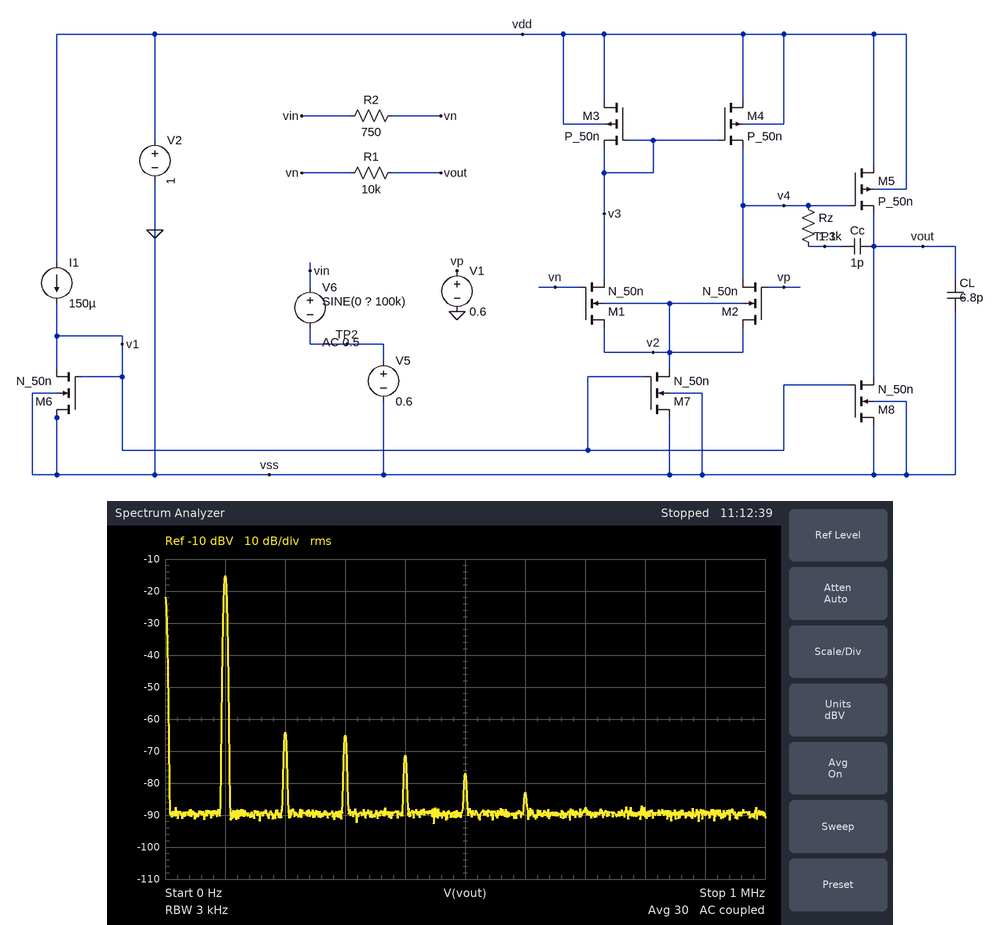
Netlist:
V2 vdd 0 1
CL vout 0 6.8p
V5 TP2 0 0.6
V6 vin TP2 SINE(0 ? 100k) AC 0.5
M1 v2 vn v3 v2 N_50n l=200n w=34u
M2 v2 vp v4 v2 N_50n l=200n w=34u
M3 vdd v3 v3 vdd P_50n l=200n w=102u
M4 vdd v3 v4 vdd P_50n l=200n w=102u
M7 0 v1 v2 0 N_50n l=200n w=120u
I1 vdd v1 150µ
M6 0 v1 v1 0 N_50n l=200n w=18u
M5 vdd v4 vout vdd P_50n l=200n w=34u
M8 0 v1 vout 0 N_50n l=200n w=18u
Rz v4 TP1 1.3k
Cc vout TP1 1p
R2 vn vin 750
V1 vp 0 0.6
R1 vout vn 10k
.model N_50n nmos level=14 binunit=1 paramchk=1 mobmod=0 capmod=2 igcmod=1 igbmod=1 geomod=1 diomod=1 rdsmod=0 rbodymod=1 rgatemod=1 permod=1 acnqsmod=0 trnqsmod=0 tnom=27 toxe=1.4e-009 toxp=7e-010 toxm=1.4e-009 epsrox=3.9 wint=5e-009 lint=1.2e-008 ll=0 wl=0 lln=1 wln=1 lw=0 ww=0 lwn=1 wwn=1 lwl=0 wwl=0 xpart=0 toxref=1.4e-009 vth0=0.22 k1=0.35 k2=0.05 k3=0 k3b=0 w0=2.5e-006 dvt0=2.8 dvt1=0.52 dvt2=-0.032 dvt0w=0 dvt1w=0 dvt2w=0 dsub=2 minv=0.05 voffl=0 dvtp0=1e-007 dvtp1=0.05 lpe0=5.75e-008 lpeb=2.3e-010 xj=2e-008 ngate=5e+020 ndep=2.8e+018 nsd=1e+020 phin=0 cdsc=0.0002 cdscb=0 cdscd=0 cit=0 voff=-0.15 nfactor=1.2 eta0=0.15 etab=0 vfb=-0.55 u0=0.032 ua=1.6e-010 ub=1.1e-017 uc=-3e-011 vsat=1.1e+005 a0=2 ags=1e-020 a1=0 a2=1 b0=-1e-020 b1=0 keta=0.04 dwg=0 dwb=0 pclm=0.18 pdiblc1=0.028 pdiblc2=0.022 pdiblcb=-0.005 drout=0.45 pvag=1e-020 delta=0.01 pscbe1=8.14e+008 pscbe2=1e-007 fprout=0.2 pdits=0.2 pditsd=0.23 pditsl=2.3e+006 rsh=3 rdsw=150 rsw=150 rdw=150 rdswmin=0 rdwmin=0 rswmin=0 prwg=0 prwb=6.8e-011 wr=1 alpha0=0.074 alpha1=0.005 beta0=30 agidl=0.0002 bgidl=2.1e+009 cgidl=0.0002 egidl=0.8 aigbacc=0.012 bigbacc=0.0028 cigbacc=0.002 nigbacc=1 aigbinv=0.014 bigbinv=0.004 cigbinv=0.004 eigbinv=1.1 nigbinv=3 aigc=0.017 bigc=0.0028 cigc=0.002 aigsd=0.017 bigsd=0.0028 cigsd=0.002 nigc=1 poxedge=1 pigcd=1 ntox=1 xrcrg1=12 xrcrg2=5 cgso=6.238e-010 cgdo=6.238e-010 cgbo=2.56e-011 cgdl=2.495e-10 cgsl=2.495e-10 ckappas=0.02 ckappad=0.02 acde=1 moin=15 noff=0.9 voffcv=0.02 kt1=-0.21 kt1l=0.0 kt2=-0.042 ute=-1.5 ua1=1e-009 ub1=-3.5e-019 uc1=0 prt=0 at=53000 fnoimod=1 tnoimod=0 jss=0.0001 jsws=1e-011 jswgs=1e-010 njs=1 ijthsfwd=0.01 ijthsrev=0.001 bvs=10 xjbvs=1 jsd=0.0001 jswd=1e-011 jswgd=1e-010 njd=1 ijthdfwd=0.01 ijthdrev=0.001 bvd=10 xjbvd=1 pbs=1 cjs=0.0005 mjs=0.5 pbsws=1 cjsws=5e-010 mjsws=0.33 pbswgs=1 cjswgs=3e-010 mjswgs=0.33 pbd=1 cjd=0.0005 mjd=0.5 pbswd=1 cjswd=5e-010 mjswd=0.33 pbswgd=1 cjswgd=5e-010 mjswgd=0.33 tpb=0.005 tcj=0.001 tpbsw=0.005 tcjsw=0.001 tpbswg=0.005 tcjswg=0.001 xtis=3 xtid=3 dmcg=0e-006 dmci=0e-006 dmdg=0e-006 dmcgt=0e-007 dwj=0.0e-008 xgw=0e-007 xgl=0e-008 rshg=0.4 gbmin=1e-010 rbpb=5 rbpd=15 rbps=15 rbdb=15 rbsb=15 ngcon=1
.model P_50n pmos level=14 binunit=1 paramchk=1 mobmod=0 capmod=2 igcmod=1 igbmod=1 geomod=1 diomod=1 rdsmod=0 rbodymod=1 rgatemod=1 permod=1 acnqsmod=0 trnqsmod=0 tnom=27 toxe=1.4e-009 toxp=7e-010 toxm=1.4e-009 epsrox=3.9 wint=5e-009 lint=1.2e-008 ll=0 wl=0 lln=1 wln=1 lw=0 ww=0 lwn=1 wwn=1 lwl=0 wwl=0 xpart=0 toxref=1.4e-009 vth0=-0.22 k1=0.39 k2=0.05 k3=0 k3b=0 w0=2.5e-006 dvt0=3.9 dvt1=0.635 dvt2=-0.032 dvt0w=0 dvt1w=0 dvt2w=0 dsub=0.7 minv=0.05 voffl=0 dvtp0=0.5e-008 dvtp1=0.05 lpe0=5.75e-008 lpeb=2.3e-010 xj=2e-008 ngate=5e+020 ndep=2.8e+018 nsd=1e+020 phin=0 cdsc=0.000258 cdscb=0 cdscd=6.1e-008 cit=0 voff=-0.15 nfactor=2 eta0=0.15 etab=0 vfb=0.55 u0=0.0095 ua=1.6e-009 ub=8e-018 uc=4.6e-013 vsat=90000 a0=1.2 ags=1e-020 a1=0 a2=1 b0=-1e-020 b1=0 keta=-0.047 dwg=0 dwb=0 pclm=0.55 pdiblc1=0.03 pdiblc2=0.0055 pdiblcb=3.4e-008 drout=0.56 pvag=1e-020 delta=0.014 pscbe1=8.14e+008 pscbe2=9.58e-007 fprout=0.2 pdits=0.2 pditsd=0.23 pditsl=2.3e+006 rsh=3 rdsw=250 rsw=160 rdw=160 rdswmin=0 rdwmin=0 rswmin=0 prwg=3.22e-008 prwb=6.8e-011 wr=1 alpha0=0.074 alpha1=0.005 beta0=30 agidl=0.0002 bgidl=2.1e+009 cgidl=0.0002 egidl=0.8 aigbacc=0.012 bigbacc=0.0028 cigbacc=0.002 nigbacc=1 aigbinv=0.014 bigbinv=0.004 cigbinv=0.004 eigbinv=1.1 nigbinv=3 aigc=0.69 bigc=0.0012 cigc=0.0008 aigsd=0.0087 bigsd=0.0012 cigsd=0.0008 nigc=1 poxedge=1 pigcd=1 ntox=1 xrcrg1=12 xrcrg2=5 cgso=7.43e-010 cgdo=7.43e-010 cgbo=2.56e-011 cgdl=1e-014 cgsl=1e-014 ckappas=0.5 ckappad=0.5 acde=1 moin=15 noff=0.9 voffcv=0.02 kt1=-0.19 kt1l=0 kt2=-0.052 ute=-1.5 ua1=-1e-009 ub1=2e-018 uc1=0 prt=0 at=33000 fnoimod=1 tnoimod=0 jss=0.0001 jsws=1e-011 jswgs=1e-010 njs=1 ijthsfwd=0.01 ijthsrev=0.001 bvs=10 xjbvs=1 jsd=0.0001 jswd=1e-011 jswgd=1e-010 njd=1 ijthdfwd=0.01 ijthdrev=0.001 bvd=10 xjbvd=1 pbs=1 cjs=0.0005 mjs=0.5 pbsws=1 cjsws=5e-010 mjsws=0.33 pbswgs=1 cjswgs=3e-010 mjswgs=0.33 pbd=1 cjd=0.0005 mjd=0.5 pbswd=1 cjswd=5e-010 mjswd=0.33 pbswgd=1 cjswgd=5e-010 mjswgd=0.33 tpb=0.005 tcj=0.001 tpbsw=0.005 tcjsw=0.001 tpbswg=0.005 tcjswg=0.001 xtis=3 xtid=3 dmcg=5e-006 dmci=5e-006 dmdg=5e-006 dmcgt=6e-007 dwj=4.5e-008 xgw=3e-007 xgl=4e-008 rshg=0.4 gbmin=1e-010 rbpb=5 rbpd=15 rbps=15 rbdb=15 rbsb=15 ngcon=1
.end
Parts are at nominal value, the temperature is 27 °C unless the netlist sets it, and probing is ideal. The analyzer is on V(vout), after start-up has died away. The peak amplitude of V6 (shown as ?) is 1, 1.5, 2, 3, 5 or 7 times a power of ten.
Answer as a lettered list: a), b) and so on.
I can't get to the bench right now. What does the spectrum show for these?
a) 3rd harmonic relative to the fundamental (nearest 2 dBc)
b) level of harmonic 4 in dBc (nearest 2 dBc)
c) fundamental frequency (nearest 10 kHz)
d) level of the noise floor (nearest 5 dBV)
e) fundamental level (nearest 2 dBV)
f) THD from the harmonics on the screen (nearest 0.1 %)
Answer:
a) -50 dBc
b) -56 dBc
c) 100 kHz
d) -90 dBV
e) -16 dBV
f) 0.5 %
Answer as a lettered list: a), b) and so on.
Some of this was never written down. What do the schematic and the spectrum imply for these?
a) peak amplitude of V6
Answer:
a) 20 mV
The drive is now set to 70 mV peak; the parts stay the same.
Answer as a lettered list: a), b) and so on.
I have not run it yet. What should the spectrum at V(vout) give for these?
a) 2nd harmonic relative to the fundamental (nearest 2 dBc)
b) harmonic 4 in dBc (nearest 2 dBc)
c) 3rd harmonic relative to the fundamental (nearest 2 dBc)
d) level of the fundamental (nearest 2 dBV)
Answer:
a) -20 dBc
b) -28 dBc
c) -14 dBc
d) -8 dBV
